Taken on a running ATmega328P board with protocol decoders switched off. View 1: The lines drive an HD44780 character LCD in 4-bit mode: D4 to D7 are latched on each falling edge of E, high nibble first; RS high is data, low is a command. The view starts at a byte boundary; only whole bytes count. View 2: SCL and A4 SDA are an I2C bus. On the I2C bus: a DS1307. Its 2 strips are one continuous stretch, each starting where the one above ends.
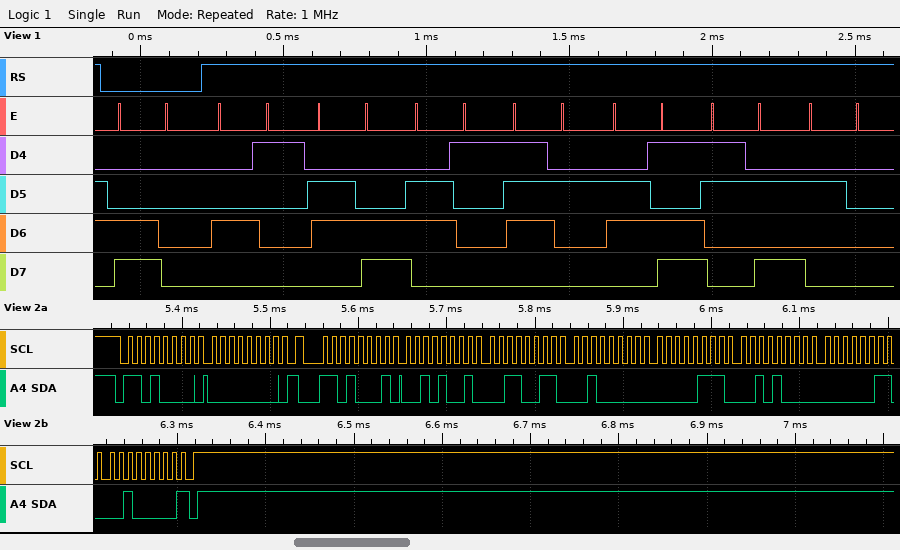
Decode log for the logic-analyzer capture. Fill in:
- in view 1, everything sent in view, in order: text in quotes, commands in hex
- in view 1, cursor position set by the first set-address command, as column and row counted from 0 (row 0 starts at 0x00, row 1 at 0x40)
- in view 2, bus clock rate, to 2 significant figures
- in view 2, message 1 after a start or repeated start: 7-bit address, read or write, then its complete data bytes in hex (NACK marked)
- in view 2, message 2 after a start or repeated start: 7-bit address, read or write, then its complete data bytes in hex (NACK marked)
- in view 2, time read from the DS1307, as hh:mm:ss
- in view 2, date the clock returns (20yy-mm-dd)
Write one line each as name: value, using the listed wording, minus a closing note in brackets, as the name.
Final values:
in view 1, everything sent in view, in order: text in quotes, commands in hex: 0xC0 "Alarm: "
in view 1, cursor position set by the first set-address command, as column and row counted from 0: column 0, row 1
in view 2, bus clock rate, to 2 significant figures: 100 kHz
in view 2, message 1 after a start or repeated start: 7-bit address, read or write, then its complete data bytes in hex: 0x68 write: 00
in view 2, message 2 after a start or repeated start: 7-bit address, read or write, then its complete data bytes in hex: 0x68 read: 29 33 20 07 28 03 20 NACK
in view 2, time read from the DS1307, as hh:mm:ss: 20:33:29
in view 2, date the clock returns: 2020-03-28
